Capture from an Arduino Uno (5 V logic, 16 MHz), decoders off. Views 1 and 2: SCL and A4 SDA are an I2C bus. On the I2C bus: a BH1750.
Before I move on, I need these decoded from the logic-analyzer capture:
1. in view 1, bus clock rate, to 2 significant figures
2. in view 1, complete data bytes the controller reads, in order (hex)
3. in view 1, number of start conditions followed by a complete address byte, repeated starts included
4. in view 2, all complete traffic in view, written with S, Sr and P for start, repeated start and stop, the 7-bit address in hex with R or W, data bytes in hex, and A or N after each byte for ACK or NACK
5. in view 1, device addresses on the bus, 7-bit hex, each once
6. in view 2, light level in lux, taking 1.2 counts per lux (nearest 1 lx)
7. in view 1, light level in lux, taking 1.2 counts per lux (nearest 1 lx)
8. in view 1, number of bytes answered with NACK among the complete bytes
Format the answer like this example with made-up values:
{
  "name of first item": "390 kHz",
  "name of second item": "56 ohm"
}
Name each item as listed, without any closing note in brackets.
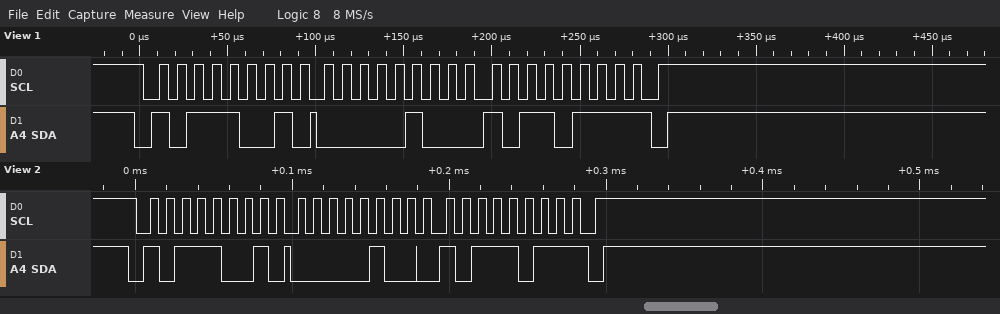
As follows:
{
  "in view 1, bus clock rate, to 2 significant figures": "100 kHz",
  "in view 1, complete data bytes the controller reads, in order": "04 B7",
  "in view 1, number of start conditions followed by a complete address byte, repeated starts included": "1",
  "in view 2, all complete traffic in view, written with S, Sr and P for start, repeated start and stop, the 7-bit address in hex with R or W, data bytes in hex, and A or N after each byte for ACK or NACK": "S 5CR A 04 A BB N P",
  "in view 1, device addresses on the bus, 7-bit hex, each once": "0x5C",
  "in view 2, light level in lux, taking 1.2 counts per lux": "1009 lx",
  "in view 1, light level in lux, taking 1.2 counts per lux": "1006 lx",
  "in view 1, number of bytes answered with NACK among the complete bytes": "1"
}
